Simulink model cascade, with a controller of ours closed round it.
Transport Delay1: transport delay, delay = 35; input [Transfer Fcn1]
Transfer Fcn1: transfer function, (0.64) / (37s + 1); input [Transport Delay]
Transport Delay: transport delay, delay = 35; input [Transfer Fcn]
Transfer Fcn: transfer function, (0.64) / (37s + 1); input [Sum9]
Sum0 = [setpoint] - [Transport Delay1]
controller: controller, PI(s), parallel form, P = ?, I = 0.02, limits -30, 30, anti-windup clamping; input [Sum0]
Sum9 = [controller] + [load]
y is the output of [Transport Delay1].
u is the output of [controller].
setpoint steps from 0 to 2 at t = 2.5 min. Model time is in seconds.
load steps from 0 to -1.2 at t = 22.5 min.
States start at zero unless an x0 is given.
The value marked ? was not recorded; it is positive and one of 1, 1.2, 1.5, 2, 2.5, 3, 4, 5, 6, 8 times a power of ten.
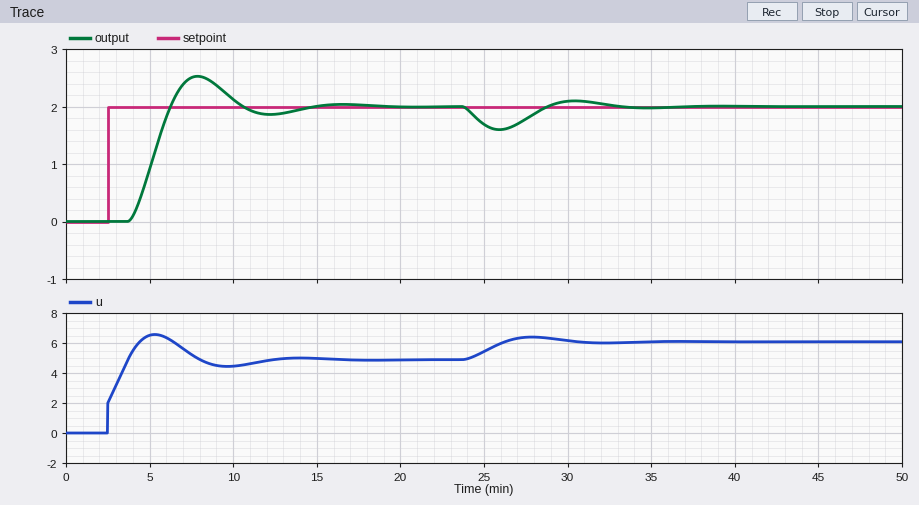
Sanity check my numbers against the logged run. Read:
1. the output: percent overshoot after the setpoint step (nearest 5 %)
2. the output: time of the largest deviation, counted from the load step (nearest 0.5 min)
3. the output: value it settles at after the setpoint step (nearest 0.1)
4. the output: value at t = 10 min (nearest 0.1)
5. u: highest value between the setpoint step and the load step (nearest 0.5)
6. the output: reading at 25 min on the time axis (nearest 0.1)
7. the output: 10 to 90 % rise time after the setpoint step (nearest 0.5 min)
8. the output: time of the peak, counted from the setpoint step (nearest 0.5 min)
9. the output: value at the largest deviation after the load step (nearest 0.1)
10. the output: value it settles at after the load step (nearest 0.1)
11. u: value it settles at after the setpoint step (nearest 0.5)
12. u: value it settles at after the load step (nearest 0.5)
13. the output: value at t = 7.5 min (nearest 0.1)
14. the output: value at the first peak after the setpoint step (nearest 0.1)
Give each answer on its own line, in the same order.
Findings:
25 %
3.5 min
2.0
2.1
6.5
1.7
2.0 min
5.5 min
1.6
2.0
5.0
6.0
2.5
2.5
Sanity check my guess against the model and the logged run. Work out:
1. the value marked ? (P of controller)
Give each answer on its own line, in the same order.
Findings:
1
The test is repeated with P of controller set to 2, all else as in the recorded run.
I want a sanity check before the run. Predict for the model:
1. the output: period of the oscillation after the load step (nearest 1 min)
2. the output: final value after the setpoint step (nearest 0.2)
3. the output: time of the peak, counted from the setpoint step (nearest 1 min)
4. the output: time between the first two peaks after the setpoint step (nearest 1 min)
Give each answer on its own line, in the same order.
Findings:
6 min
2.0
4 min
6 min
